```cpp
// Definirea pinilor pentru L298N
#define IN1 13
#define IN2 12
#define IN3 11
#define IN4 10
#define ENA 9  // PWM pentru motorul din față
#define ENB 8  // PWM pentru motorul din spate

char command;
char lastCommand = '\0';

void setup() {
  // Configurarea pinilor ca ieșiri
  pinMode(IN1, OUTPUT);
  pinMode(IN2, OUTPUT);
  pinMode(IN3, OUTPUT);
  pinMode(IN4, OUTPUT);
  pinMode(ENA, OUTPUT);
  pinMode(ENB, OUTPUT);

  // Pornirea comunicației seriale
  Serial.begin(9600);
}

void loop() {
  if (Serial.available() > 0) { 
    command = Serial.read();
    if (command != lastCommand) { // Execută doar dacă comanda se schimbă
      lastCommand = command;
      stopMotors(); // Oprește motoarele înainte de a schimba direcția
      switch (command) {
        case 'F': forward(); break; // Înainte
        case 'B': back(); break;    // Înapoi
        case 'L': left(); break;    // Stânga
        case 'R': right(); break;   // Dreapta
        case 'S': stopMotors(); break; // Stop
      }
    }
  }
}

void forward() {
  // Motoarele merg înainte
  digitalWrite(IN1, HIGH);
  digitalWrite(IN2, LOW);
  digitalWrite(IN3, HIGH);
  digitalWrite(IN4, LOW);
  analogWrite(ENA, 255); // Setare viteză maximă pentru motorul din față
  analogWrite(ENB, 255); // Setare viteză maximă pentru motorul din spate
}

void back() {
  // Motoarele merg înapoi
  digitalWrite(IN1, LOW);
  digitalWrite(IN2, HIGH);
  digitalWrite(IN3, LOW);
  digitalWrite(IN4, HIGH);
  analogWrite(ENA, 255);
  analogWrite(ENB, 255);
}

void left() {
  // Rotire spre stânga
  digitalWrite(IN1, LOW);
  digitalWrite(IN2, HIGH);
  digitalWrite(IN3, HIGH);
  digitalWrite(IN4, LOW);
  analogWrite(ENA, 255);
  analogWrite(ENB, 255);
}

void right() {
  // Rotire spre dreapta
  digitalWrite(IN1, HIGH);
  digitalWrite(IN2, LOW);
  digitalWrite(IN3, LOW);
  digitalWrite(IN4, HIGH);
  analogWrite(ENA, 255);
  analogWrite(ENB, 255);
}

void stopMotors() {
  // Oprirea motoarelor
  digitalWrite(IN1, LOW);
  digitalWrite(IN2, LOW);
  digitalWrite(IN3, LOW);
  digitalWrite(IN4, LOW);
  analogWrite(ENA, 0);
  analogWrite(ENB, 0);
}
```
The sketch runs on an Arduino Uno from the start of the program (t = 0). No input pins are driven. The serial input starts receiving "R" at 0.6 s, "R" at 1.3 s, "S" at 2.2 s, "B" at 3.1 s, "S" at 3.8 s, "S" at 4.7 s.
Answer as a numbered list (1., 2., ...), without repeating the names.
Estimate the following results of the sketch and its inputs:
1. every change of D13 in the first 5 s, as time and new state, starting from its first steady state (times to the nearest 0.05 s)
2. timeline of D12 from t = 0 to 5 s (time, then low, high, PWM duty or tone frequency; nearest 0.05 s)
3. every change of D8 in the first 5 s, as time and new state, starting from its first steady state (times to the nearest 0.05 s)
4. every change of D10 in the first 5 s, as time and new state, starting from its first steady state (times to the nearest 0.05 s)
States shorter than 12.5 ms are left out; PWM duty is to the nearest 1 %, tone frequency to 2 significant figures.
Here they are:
1. 0 s low; 0.6 s high; 2.2 s low
2. 0 s low; 3.1 s high; 3.8 s low
3. 0 s low; 0.6 s high; 2.2 s low; 3.1 s high; 3.8 s low
4. 0 s low; 0.6 s high; 2.2 s low; 3.1 s high; 3.8 s low
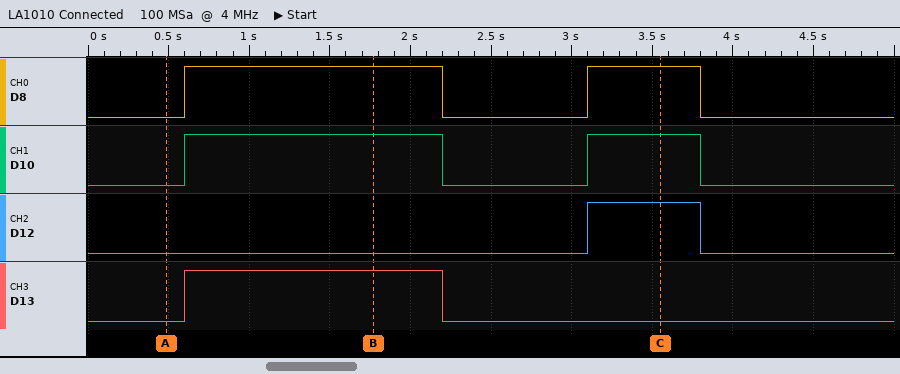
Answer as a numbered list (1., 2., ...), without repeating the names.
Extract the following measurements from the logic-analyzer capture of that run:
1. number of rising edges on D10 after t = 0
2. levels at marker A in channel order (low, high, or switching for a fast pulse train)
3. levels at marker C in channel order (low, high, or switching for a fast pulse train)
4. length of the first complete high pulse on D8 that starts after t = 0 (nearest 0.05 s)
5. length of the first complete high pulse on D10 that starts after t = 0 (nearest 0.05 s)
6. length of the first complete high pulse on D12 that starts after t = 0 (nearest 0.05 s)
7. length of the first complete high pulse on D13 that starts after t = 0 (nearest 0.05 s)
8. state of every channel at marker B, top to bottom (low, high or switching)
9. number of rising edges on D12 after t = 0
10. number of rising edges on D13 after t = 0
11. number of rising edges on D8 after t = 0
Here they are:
1. 2
2. D8 low, D10 low, D12 low, D13 low
3. D8 high, D10 high, D12 high, D13 low
4. 1.60 s
5. 1.60 s
6. 0.70 s
7. 1.60 s
8. D8 high, D10 high, D12 low, D13 high
9. 1
10. 1
11. 2
